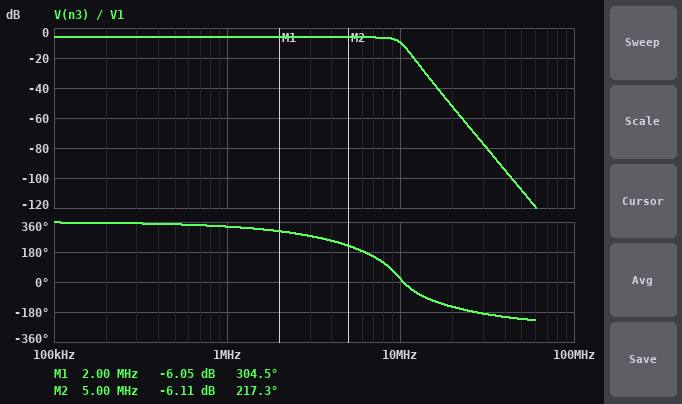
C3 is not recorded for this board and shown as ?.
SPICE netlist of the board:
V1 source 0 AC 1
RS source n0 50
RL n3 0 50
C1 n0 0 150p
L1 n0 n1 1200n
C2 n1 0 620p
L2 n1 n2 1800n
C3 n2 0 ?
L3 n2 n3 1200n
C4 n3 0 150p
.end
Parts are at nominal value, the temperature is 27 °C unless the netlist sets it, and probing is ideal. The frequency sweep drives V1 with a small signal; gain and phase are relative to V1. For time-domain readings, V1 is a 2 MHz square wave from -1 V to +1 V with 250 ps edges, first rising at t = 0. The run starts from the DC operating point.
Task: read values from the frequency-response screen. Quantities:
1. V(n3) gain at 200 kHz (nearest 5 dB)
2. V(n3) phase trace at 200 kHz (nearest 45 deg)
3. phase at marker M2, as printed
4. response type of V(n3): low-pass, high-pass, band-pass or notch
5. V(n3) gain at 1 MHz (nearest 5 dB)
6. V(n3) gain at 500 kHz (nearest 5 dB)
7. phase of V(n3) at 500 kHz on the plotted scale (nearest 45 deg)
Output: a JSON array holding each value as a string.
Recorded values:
["-5 dB", "360 deg", "217.3 deg", "low-pass", "-5 dB", "-5 dB", "360 deg"]
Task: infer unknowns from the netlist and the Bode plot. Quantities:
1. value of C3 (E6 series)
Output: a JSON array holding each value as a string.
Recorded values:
["470 pF"]
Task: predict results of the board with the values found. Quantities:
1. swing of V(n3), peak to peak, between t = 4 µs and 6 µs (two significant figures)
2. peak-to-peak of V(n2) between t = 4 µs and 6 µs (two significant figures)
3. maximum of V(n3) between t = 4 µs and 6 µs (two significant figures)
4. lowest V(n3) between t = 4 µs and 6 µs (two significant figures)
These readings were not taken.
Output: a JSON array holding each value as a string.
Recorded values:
["1.3 V", "1.5 V", "660 mV", "-660 mV"]
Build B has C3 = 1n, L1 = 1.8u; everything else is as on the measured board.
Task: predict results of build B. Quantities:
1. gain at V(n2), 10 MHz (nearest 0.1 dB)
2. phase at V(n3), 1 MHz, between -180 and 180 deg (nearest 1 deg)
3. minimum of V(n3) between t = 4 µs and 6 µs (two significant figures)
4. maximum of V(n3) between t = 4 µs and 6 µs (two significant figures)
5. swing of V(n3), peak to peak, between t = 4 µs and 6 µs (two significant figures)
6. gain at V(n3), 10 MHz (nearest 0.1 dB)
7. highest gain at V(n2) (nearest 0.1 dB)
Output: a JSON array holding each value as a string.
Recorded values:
["-20.8 dB", "-35 deg", "-600 mV", "600 mV", "1.2 V", "-24.5 dB", "-4.8 dB"]
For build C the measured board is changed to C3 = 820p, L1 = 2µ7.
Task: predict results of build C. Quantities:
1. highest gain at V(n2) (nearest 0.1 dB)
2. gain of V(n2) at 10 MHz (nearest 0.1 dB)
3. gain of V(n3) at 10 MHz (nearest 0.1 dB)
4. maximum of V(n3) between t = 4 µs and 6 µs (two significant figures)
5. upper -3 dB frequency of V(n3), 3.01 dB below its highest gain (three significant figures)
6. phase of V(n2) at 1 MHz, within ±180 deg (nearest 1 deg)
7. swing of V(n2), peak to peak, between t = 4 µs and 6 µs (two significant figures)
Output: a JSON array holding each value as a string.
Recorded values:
["-4.5 dB", "-22.7 dB", "-26.4 dB", "580 mV", "7.78 MHz", "-28 deg", "1.2 V"]
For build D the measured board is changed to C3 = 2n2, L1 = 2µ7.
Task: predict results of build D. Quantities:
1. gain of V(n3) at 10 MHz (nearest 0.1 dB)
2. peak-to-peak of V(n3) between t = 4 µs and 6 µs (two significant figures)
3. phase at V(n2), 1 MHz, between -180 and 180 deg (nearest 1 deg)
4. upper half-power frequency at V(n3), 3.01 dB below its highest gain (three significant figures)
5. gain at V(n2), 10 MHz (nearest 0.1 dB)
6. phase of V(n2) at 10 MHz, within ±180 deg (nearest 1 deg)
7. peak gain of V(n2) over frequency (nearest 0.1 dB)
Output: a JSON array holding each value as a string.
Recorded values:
["-38.3 dB", "1.1 V", "-41 deg", "2.68 MHz", "-34.6 dB", "-2 deg", "-6.0 dB"]
